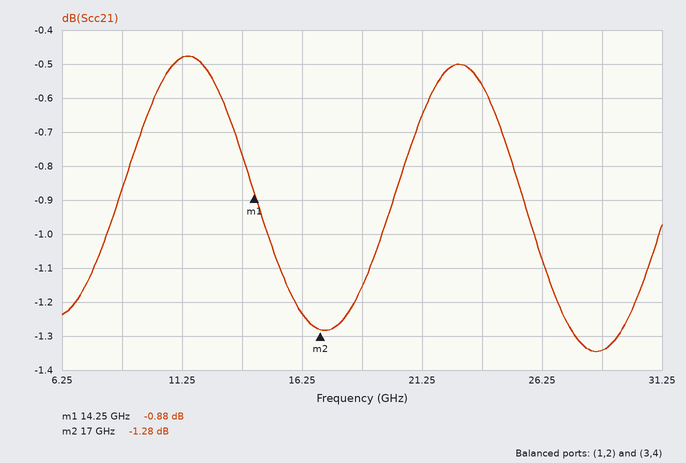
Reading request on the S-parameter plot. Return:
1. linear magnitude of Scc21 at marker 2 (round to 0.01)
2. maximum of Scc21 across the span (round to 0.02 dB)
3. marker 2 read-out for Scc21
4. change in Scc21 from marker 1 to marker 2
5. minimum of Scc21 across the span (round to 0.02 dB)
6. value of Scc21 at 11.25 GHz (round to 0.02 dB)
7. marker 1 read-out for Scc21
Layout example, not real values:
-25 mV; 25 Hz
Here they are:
0.86; -0.48 dB; -1.28 dB; -0.40 dB; -1.34 dB; -0.48 dB; -0.88 dB
